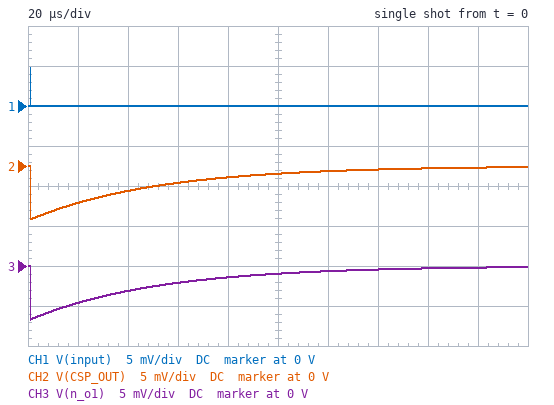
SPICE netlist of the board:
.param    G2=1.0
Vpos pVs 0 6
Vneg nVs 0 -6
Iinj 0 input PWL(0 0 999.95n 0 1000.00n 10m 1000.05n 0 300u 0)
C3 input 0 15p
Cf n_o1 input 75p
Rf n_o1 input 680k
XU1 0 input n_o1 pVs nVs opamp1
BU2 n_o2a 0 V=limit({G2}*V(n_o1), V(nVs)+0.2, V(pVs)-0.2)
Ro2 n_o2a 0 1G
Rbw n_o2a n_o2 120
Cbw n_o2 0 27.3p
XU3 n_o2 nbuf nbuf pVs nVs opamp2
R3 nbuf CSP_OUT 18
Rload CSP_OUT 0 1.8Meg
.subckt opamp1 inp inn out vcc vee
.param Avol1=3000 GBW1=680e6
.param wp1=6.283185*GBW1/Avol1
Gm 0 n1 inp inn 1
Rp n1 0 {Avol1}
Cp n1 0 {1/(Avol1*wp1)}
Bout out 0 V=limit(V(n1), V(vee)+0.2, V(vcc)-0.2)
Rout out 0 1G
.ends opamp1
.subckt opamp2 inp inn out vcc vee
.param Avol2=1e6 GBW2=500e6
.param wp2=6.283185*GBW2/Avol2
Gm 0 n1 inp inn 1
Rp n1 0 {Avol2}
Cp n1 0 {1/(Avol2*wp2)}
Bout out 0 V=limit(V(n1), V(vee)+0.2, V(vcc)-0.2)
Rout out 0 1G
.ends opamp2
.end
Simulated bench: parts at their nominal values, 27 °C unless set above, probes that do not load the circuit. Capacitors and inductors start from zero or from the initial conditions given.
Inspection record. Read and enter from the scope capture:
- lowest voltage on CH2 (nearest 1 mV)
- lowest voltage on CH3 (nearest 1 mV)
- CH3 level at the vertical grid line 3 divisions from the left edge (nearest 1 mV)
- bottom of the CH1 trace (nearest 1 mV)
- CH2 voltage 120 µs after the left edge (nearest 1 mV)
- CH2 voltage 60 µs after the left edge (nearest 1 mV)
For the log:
-7 mV
-7 mV
-2 mV
0 V
-1 mV
-2 mV
